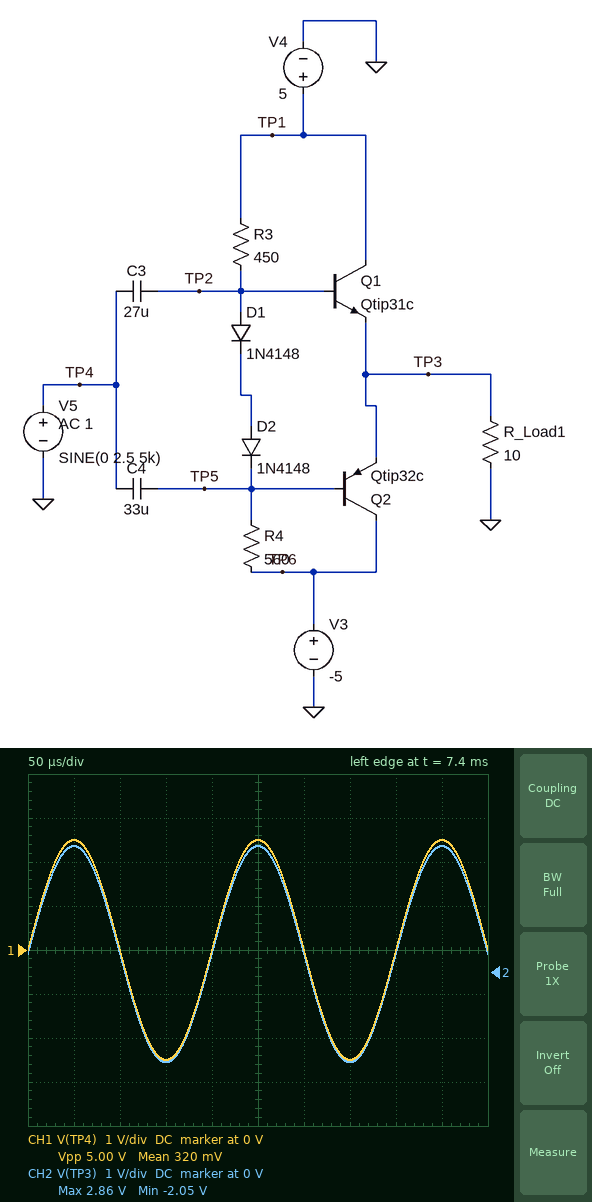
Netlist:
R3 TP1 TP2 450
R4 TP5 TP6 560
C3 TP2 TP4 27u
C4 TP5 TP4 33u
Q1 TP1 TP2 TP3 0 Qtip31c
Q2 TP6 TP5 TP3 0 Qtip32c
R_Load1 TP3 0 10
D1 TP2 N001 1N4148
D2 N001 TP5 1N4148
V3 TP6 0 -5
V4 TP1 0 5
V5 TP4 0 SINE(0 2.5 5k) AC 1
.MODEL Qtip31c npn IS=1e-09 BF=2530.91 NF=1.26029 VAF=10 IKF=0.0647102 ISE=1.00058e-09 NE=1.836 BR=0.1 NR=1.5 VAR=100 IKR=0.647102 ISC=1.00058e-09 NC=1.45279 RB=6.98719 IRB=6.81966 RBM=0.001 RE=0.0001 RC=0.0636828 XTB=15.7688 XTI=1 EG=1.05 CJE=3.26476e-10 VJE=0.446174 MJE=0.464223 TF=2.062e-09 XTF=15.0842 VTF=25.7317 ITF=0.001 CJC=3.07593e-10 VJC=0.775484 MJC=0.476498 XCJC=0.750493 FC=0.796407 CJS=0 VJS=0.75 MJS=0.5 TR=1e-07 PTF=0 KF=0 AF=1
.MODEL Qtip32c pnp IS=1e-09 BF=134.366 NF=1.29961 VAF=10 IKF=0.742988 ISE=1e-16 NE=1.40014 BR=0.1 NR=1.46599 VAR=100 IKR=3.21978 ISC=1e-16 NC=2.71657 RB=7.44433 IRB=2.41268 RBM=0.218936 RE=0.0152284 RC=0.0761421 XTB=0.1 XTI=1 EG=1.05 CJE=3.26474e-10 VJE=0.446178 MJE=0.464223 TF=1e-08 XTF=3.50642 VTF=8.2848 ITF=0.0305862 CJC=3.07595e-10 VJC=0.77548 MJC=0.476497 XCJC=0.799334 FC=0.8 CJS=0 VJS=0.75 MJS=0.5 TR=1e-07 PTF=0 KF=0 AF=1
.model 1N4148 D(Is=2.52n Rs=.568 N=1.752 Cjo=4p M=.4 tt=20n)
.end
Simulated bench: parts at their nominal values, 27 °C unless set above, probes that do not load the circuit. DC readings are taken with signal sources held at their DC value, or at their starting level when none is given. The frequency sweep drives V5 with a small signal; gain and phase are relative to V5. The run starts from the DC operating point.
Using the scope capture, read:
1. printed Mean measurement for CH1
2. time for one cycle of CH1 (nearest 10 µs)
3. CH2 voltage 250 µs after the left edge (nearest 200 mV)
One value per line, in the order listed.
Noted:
320 mV
200 µs
2.8 V
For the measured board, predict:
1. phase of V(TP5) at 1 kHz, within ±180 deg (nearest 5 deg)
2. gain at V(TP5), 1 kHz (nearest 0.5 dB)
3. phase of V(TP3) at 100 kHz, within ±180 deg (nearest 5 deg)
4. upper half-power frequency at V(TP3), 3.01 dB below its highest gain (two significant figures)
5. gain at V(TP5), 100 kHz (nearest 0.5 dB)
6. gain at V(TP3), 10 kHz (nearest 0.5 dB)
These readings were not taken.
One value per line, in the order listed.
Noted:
0 deg
0 dB
0 deg
23 MHz
0 dB
0 dB
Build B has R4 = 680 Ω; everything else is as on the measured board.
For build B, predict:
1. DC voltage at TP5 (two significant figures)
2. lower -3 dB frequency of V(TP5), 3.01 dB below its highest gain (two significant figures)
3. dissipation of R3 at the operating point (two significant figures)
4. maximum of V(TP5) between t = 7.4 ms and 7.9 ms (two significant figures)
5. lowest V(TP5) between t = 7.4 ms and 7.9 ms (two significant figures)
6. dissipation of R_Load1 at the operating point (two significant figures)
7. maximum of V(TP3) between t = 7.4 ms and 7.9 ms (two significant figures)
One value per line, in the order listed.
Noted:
73 mV
12 Hz
29 mW
2.6 V
-2.4 V
53 mW
3.2 V
